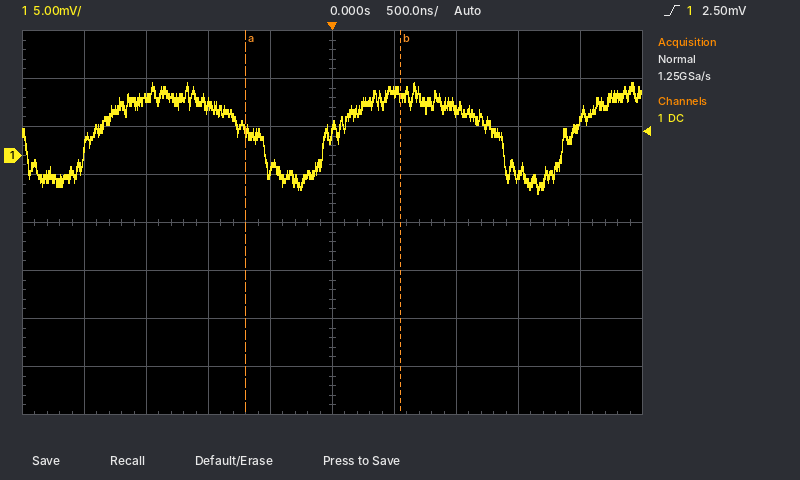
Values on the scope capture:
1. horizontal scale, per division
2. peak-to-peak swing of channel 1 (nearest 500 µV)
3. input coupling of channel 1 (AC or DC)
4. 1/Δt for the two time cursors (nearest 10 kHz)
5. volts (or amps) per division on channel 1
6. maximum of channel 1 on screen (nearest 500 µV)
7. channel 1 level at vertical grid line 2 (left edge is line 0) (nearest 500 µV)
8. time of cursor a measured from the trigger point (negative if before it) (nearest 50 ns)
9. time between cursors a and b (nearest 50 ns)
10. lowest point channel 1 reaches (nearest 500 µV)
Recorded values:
500 ns
11.5 mV
DC
800 kHz
5 mV
7.5 mV
6.0 mV
-700 ns
1.25 µs
-4.0 mV
